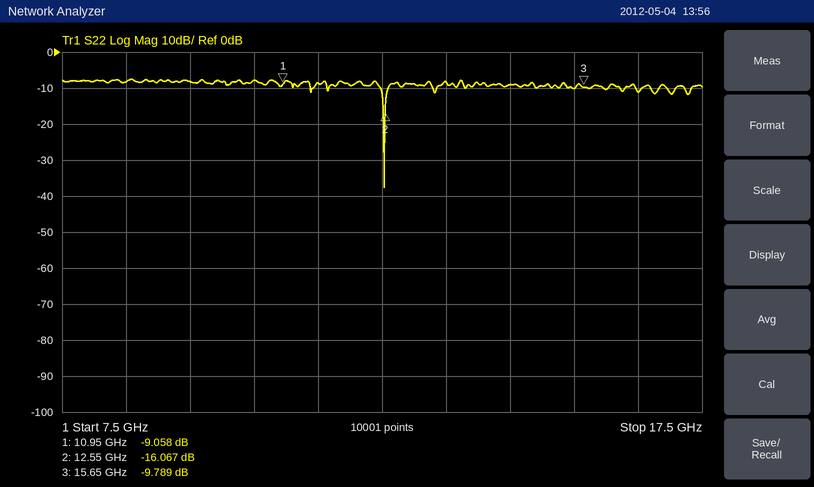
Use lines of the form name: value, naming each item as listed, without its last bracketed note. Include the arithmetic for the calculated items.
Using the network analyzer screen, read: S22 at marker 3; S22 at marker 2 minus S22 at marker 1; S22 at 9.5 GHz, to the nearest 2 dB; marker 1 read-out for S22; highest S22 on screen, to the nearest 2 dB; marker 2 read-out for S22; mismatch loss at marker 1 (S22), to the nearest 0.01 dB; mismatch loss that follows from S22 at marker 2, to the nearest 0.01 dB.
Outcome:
S22 at marker 3: -9.789 dB
S22 at marker 2 minus S22 at marker 1: -16.067 − (-9.058) = -7.009 dB
S22 at 9.5 GHz, to the nearest 2 dB: -8 dB
marker 1 read-out for S22: -9.058 dB
highest S22 on screen, to the nearest 2 dB: -8 dB
marker 2 read-out for S22: -16.067 dB
mismatch loss at marker 1 (S22), to the nearest 0.01 dB: −10 log10(1 − 10^(-9.058/10)) ≈ 0.58 dB
mismatch loss that follows from S22 at marker 2, to the nearest 0.01 dB: −10 log10(1 − 10^(-16.067/10)) ≈ 0.11 dB
